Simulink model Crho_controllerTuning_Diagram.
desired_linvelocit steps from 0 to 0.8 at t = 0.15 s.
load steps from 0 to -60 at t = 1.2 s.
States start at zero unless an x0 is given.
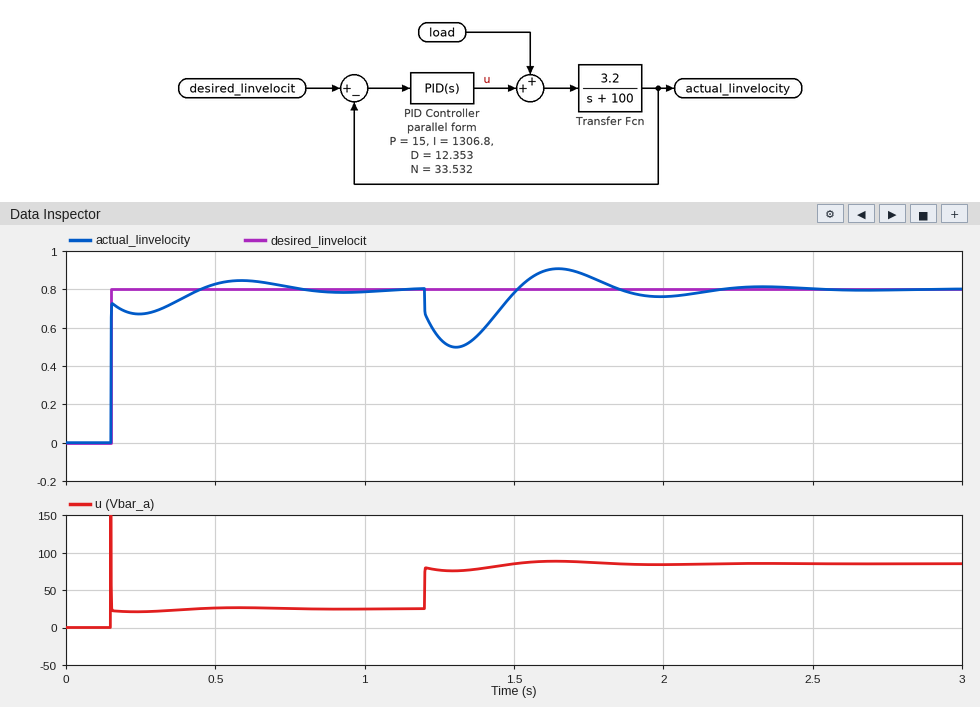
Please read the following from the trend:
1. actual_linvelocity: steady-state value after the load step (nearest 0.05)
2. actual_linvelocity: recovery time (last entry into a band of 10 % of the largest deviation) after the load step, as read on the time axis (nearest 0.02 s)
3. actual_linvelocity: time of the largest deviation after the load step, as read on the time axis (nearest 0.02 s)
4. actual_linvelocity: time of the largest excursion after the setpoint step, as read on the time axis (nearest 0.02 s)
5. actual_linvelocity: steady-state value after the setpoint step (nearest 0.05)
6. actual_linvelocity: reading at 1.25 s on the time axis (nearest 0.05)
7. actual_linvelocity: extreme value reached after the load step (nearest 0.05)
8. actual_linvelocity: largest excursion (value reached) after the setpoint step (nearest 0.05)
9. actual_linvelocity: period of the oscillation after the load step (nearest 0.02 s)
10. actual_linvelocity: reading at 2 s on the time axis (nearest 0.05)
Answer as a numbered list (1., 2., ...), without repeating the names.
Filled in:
1. 0.80
2. 2.06 s
3. 1.30 s
4. 0.58 s
5. 0.80
6. 0.55
7. 0.50
8. 0.85
9. 0.68 s
10. 0.75
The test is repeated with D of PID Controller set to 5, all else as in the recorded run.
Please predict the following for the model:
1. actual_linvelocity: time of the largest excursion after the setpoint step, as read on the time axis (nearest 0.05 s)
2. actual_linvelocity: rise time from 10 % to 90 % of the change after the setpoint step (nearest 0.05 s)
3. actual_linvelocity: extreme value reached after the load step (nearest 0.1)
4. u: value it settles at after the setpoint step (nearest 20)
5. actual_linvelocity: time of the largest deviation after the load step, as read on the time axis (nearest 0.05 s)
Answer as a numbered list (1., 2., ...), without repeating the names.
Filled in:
1. 0.45 s
2. 0.15 s
3. 0.4
4. 20
5. 1.25 s
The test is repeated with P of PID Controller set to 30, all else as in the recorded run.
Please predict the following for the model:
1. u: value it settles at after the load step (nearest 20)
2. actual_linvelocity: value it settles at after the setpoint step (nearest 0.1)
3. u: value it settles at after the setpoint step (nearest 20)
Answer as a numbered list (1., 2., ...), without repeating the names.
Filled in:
1. 80
2. 0.8
3. 20
